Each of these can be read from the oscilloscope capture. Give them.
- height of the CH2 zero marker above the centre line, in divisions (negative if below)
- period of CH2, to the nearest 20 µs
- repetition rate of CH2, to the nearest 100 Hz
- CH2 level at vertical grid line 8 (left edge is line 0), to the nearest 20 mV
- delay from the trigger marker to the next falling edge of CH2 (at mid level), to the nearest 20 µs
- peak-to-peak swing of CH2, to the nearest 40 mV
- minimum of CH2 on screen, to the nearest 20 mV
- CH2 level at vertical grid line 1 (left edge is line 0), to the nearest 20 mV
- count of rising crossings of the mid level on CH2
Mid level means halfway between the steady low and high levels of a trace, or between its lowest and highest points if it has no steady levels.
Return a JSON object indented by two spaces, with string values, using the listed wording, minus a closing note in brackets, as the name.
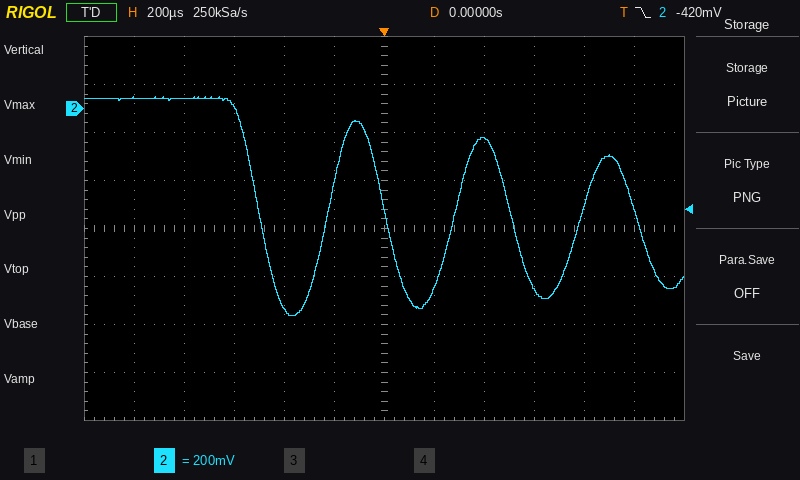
{
  "height of the CH2 zero marker above the centre line, in divisions": "+2.5 div",
  "period of CH2, to the nearest 20 µs": "500 µs",
  "repetition rate of CH2, to the nearest 100 Hz": "2.0 kHz",
  "CH2 level at vertical grid line 8 (left edge is line 0), to the nearest 20 mV": "-120 mV",
  "delay from the trigger marker to the next falling edge of CH2 (at mid level), to the nearest 20 µs": "500 µs",
  "peak-to-peak swing of CH2, to the nearest 40 mV": "920 mV",
  "minimum of CH2 on screen, to the nearest 20 mV": "-860 mV",
  "CH2 level at vertical grid line 1 (left edge is line 0), to the nearest 20 mV": "40 mV",
  "count of rising crossings of the mid level on CH2": "3"
}
